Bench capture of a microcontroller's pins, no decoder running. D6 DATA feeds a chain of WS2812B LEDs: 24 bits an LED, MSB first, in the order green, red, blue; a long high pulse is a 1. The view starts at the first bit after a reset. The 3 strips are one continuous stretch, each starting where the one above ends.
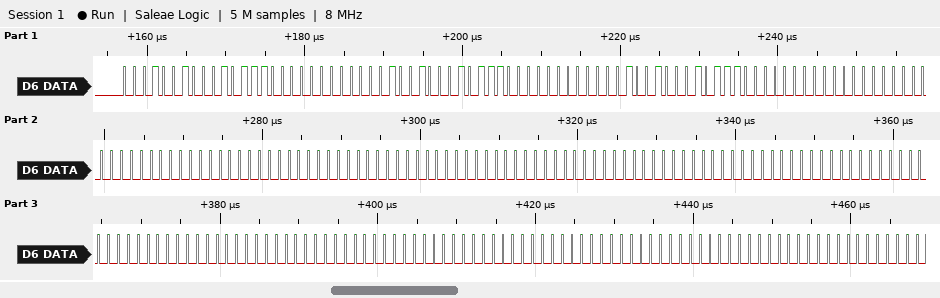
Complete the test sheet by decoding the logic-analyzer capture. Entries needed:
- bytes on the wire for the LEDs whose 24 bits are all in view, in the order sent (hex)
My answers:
12 2E 00 12 2E 00 12 2E 00 00 00 00 00 00 00 00 00 00 00 00 00 00 00 00 00 00 00 00 00 00
